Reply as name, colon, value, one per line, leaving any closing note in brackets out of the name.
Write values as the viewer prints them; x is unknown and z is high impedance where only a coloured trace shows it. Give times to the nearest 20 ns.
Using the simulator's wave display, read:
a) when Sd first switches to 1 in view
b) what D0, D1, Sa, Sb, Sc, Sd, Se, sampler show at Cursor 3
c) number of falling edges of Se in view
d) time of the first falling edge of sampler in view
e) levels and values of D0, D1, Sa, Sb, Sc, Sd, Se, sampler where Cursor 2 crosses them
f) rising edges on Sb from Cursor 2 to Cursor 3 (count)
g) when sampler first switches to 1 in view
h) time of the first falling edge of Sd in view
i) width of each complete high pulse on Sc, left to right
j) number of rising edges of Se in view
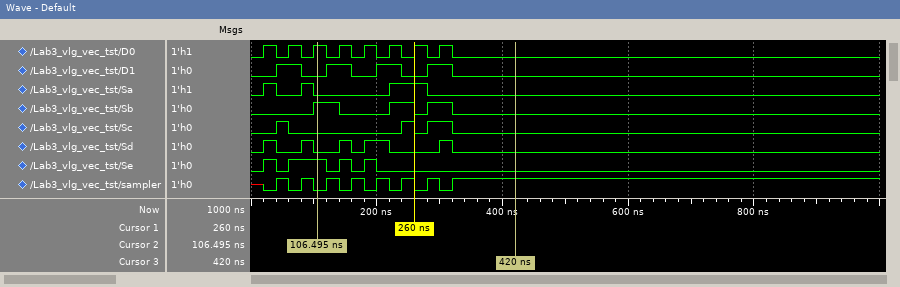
when Sd first switches to 1 in view: 20 ns
what D0, D1, Sa, Sb, Sc, Sd, Se, sampler show at Cursor 3: D0=0, D1=0, Sa=0, Sb=0, Sc=0, Sd=0, Se=0, sampler=1
number of falling edges of Se in view: 4
time of the first falling edge of sampler in view: 60 ns
levels and values of D0, D1, Sa, Sb, Sc, Sd, Se, sampler where Cursor 2 crosses them: D0=1, D1=0, Sa=0, Sb=1, Sc=0, Sd=0, Se=1, sampler=0
rising edges on Sb from Cursor 2 to Cursor 3: 2
when sampler first switches to 1 in view: 40 ns
time of the first falling edge of Sd in view: 40 ns
width of each complete high pulse on Sc, left to right: 20 ns, 20 ns, 40 ns
number of rising edges of Se in view: 4
